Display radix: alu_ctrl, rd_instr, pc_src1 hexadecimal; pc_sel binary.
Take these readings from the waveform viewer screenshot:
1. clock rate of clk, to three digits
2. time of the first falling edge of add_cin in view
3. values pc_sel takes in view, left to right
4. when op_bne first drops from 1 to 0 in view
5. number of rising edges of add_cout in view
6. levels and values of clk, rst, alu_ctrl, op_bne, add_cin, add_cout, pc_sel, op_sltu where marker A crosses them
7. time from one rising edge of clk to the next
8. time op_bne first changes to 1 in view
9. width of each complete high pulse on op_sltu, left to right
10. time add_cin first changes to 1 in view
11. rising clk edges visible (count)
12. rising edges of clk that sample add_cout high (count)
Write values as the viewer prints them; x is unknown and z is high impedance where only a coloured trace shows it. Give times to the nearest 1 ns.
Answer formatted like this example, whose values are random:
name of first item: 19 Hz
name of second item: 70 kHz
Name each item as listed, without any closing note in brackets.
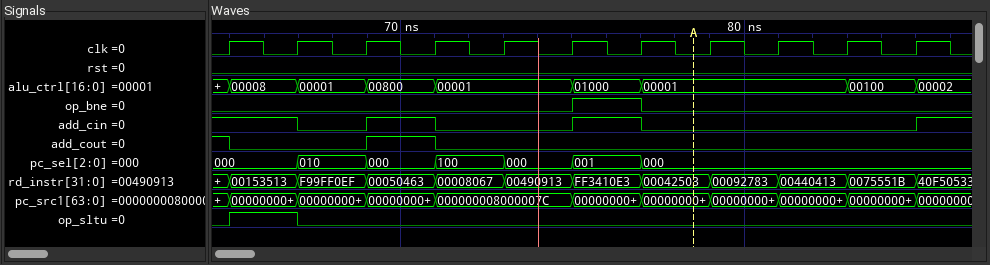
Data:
clock rate of clk, to three digits: 500 MHz
time of the first falling edge of add_cin in view: 67 ns
values pc_sel takes in view, left to right: 000, 010, 000, 100, 000, 001, 000
when op_bne first drops from 1 to 0 in view: 77 ns
number of rising edges of add_cout in view: 1
levels and values of clk, rst, alu_ctrl, op_bne, add_cin, add_cout, pc_sel, op_sltu where marker A crosses them: clk=0, rst=0, alu_ctrl=00001, op_bne=0, add_cin=0, add_cout=0, pc_sel=000, op_sltu=0
time from one rising edge of clk to the next: 2 ns
time op_bne first changes to 1 in view: 75 ns
width of each complete high pulse on op_sltu, left to right: 2 ns
time add_cin first changes to 1 in view: 69 ns
rising clk edges visible: 11
rising edges of clk that sample add_cout high: 2
